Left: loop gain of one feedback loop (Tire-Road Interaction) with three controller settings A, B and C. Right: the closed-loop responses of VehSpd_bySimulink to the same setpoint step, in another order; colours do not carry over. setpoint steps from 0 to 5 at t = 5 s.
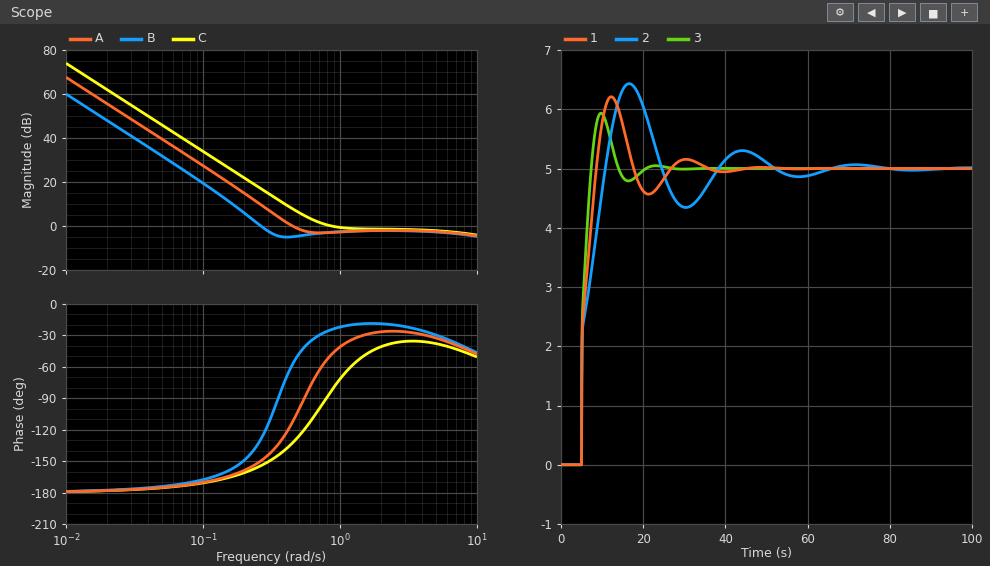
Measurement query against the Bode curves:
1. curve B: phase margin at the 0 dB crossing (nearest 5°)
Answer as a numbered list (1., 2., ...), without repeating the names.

1. 50°
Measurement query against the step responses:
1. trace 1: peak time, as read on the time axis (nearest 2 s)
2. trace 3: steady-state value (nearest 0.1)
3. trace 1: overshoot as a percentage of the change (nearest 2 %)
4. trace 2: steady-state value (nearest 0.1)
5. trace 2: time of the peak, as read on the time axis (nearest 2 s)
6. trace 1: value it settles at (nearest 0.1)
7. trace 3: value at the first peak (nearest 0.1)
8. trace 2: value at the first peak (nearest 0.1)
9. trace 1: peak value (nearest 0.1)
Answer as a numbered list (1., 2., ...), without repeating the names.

1. 12 s
2. 5.0
3. 24 %
4. 5.0
5. 16 s
6. 5.0
7. 5.9
8. 6.4
9. 6.2
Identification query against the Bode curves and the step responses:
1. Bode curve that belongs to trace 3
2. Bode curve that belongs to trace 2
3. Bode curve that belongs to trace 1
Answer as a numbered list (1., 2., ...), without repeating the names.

1. C
2. B
3. A
